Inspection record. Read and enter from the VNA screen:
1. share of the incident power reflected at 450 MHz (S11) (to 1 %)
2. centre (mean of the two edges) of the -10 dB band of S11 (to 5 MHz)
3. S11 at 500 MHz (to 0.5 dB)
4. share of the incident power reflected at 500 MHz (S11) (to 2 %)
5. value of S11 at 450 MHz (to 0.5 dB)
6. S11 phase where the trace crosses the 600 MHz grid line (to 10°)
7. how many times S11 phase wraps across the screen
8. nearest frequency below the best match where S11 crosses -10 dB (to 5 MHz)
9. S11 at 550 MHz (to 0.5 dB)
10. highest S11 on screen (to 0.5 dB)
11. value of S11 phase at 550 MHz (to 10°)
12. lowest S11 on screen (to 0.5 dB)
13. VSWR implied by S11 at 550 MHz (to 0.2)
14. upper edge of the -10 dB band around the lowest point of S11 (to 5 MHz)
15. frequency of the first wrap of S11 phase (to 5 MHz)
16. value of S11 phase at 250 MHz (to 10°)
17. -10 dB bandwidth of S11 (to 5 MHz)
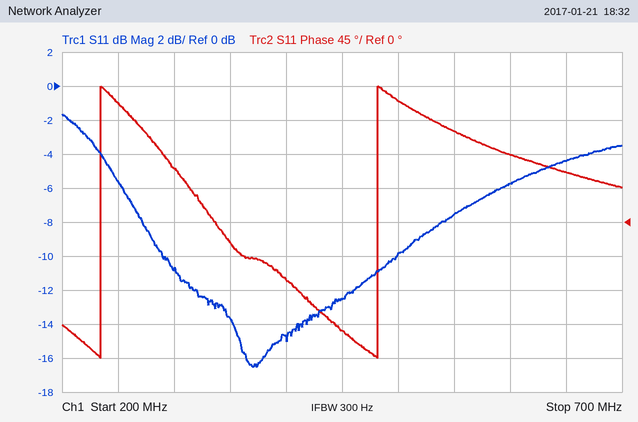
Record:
6 %
395 MHz
-10.0 dB
10 %
-12.5 dB
90°
2
290 MHz
-7.5 dB
-1.5 dB
120°
-16.5 dB
2.4
500 MHz
235 MHz
160°
210 MHz
